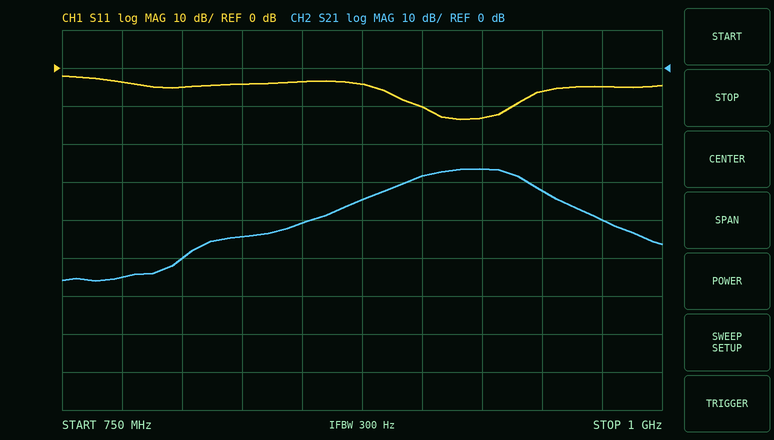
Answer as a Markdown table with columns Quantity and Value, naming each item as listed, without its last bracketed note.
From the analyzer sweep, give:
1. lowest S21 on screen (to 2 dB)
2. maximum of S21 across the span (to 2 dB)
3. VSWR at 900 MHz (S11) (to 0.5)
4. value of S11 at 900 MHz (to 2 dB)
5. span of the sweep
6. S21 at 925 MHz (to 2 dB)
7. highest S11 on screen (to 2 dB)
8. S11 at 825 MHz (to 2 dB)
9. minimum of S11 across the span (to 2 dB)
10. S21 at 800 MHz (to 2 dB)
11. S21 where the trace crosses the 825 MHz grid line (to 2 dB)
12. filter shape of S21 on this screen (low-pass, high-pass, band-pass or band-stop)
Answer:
| Quantity | Value |
|---|---|
| lowest S21 on screen | -56 dB |
| maximum of S21 across the span | -26 dB |
| VSWR at 900 MHz (S11) | 2.0 |
| value of S11 at 900 MHz | -10 dB |
| span of the sweep | 250 MHz |
| S21 at 925 MHz | -26 dB |
| highest S11 on screen | -2 dB |
| S11 at 825 MHz | -4 dB |
| minimum of S11 across the span | -14 dB |
| S21 at 800 MHz | -50 dB |
| S21 where the trace crosses the 825 MHz grid line | -44 dB |
| filter shape of S21 on this screen | band-pass |
